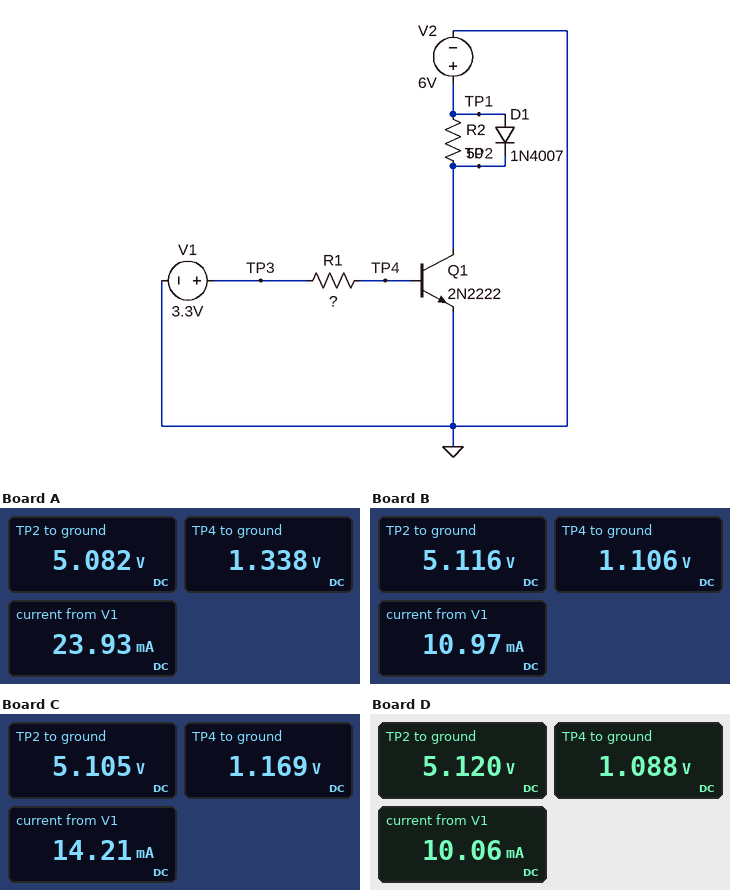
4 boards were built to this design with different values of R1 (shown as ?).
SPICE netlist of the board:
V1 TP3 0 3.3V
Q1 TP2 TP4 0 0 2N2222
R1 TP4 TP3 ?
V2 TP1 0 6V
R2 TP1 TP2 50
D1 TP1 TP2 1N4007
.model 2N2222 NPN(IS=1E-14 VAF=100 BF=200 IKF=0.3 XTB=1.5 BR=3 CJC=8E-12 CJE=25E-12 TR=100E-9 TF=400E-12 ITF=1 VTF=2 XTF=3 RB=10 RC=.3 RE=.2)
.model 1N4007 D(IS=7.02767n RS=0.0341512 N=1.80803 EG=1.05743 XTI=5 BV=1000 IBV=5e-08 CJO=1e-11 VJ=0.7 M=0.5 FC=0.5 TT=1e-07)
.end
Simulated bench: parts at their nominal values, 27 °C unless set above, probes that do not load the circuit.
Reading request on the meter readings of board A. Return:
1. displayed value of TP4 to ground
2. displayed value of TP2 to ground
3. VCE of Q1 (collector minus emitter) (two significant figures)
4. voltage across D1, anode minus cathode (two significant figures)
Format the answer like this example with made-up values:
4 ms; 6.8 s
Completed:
1.338 V; 5.082 V; 5.1 V; 920 mV
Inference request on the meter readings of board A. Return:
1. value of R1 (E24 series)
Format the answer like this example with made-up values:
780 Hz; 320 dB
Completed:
82 Ω
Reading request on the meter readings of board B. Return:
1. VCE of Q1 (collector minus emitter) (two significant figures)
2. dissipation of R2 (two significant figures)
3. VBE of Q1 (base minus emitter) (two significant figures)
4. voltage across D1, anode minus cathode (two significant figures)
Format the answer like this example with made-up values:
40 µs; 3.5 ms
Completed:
5.1 V; 16 mW; 1.1 V; 880 mV
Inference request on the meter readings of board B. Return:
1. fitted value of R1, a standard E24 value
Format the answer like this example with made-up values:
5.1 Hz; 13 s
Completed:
200 Ω
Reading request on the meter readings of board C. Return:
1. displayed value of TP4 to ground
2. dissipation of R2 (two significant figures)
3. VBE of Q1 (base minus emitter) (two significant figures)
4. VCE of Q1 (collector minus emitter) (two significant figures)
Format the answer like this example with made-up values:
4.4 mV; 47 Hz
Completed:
1.169 V; 16 mW; 1.2 V; 5.1 V
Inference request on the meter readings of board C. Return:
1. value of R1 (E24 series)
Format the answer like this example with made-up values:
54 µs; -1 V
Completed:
150 Ω
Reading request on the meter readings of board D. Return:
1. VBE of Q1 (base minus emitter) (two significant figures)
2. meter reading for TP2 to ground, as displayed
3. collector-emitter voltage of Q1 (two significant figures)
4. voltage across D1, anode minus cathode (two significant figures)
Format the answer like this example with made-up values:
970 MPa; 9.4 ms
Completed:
1.1 V; 5.120 V; 5.1 V; 880 mV
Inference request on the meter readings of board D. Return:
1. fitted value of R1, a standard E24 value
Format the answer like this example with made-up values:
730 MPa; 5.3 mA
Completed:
220 Ω
